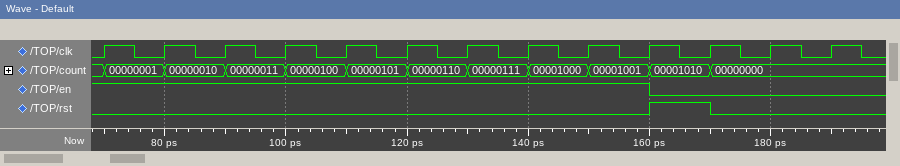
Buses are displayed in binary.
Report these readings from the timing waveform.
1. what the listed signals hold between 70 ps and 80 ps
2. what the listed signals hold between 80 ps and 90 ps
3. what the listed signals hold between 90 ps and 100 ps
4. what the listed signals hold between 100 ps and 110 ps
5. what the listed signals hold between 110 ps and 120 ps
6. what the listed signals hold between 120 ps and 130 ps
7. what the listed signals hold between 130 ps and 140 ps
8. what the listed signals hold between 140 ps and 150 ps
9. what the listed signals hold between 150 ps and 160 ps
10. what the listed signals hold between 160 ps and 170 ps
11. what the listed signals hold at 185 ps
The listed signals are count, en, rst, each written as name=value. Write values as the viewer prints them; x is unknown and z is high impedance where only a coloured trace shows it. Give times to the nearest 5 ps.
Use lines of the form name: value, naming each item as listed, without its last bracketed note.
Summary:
what the listed signals hold between 70 ps and 80 ps: count=00000001, en=1, rst=0
what the listed signals hold between 80 ps and 90 ps: count=00000010, en=1, rst=0
what the listed signals hold between 90 ps and 100 ps: count=00000011, en=1, rst=0
what the listed signals hold between 100 ps and 110 ps: count=00000100, en=1, rst=0
what the listed signals hold between 110 ps and 120 ps: count=00000101, en=1, rst=0
what the listed signals hold between 120 ps and 130 ps: count=00000110, en=1, rst=0
what the listed signals hold between 130 ps and 140 ps: count=00000111, en=1, rst=0
what the listed signals hold between 140 ps and 150 ps: count=00001000, en=1, rst=0
what the listed signals hold between 150 ps and 160 ps: count=00001001, en=1, rst=0
what the listed signals hold between 160 ps and 170 ps: count=00001010, en=0, rst=1
what the listed signals hold at 185 ps: count=00000000, en=0, rst=0
